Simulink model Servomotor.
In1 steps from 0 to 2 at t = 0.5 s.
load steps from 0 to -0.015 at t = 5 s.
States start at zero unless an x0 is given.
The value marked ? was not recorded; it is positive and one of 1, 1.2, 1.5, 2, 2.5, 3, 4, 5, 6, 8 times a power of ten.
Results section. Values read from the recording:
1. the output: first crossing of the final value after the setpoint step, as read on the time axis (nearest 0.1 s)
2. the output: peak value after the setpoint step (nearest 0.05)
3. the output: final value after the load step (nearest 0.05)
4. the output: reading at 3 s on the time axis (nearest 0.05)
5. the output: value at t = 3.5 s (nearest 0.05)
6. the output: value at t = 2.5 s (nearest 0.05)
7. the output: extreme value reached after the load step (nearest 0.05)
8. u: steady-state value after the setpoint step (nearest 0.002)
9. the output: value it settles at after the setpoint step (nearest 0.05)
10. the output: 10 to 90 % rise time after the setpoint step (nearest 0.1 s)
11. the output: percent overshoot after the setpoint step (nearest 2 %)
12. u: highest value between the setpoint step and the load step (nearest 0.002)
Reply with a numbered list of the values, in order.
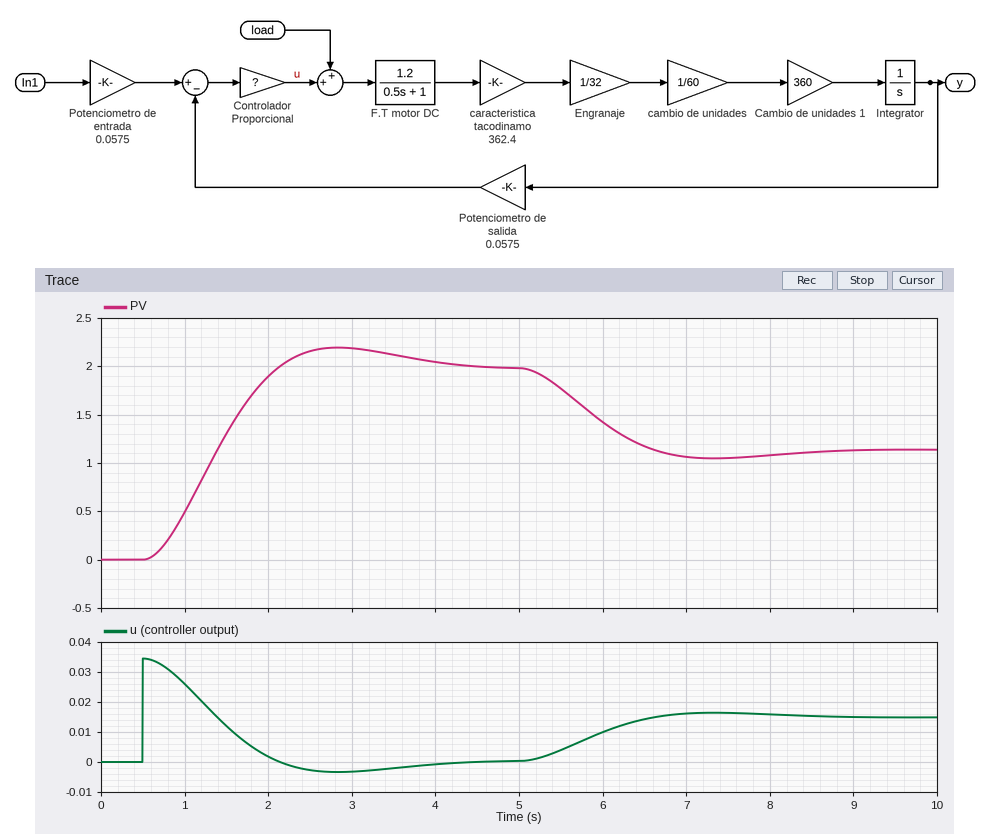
1. 2.1 s
2. 2.20
3. 1.15
4. 2.20
5. 2.10
6. 2.15
7. 1.05
8. 0.000
9. 2.00
10. 1.1 s
11. 10 %
12. 0.034
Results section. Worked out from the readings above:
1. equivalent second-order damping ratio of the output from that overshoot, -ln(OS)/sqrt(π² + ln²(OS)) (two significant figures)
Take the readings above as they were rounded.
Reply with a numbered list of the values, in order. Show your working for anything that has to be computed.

1. ln(0.1) = -2.303; 2.303 / sqrt(9.870 + 5.302) = 0.59
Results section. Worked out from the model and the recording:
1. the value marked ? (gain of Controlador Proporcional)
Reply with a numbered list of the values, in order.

1. 0.3
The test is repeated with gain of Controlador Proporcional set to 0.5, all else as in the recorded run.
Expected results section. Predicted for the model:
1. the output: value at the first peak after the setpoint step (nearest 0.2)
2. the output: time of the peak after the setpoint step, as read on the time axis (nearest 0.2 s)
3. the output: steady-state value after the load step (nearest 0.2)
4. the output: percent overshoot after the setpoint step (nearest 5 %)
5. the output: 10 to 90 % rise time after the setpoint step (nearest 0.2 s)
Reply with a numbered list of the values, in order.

1. 2.4
2. 2.2 s
3. 1.4
4. 20 %
5. 0.8 s
